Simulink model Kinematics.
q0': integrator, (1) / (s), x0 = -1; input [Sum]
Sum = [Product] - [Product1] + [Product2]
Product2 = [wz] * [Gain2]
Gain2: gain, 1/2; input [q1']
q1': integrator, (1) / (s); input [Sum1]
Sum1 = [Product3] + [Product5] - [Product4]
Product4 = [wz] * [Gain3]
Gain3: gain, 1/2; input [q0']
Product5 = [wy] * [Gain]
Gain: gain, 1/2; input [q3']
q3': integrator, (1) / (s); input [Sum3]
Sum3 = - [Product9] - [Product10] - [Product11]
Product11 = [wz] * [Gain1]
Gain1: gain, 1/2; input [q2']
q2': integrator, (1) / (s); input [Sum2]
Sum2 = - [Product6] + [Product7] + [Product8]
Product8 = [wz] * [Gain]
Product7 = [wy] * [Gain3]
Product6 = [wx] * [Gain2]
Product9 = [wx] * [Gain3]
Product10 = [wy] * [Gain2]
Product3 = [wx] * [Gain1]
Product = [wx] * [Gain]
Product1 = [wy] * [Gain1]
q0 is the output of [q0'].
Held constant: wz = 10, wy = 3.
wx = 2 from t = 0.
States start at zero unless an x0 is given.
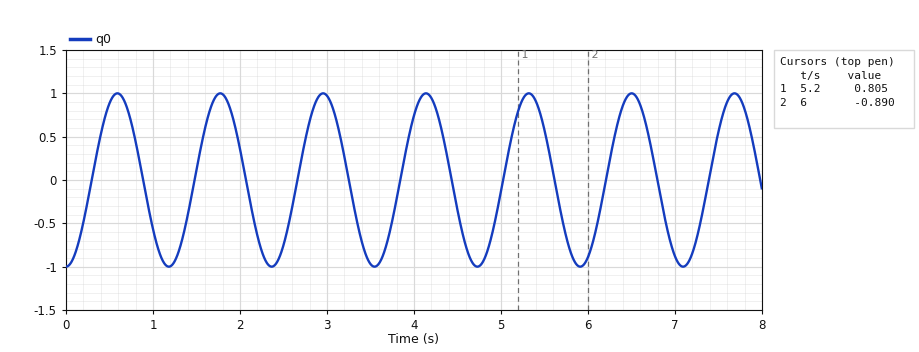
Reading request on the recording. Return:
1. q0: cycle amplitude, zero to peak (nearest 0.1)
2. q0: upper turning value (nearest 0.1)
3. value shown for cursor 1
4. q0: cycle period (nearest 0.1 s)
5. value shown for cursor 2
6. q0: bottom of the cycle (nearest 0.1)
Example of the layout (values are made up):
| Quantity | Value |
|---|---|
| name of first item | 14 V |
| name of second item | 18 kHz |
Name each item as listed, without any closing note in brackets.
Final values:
| Quantity | Value |
|---|---|
| q0: cycle amplitude, zero to peak | 1.0 |
| q0: upper turning value | 1.0 |
| value shown for cursor 1 | 0.805 |
| q0: cycle period | 1.2 s |
| value shown for cursor 2 | -0.890 |
| q0: bottom of the cycle | -1.0 |
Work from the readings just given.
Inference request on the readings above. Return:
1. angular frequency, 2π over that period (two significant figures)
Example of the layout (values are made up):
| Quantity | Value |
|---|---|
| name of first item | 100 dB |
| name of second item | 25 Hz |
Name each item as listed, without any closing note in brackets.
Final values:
| Quantity | Value |
|---|---|
| angular frequency, 2π over that period | 5.2 rad/s |
